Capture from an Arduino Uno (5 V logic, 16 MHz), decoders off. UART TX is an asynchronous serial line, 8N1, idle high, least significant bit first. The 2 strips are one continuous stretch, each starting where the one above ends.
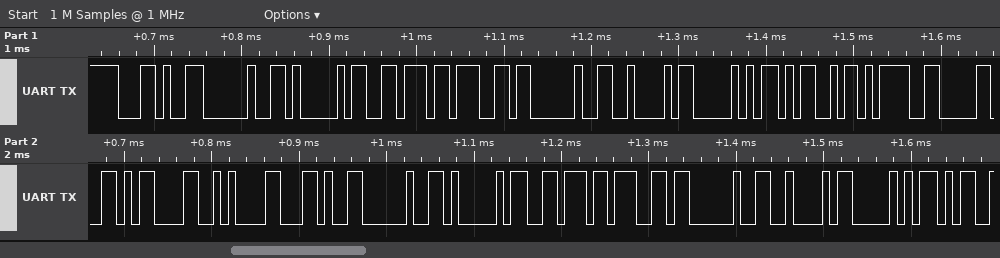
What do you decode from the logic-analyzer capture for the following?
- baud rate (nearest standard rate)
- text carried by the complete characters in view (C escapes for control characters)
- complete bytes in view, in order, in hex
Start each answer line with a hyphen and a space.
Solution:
- 115200 baud
- ", Avg BPM=0\r\n, Avg BP"
- 2C 20 41 76 67 20 42 50 4D 3D 30 0D 0A 2C 20 41 76 67 20 42 50
